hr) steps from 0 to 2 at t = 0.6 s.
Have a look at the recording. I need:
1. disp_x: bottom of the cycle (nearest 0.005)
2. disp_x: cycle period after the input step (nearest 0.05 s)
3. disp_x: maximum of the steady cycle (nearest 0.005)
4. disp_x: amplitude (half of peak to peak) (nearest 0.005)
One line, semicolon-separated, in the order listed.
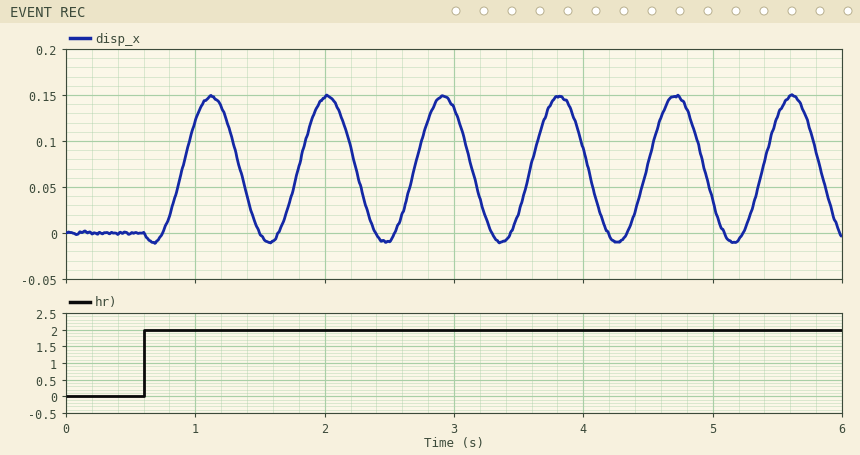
-0.010; 0.90 s; 0.150; 0.080
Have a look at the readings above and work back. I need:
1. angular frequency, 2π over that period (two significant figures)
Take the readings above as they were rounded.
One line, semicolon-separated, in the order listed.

7.0 rad/s
